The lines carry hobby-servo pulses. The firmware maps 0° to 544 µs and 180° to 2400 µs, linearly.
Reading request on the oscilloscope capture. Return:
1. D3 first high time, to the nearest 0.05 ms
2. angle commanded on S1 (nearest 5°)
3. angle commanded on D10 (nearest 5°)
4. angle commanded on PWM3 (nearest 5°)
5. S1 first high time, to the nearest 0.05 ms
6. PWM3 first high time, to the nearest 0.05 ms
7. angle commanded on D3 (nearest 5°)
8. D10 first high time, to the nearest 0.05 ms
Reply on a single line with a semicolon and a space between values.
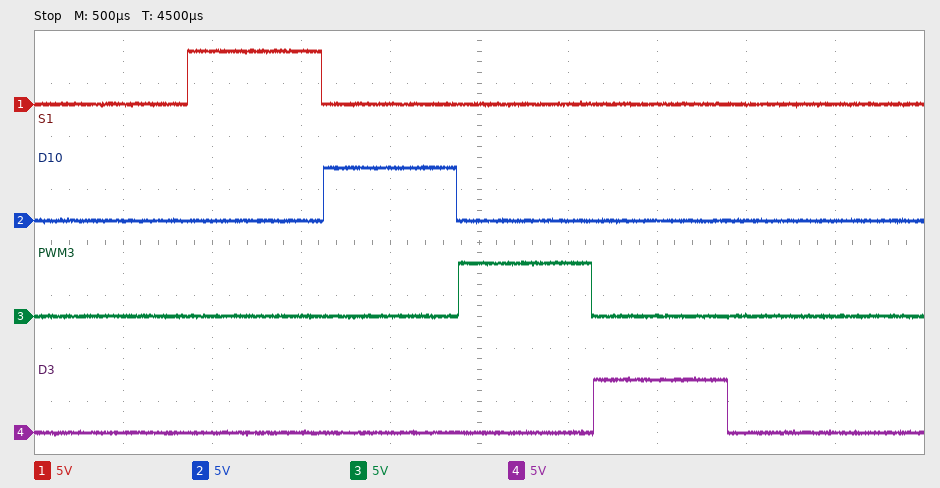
0.75 ms; 20°; 20°; 20°; 0.75 ms; 0.75 ms; 20°; 0.75 ms
